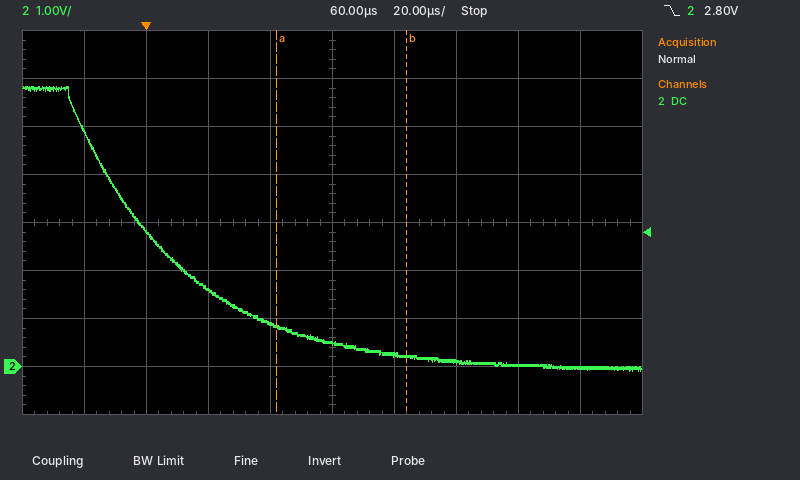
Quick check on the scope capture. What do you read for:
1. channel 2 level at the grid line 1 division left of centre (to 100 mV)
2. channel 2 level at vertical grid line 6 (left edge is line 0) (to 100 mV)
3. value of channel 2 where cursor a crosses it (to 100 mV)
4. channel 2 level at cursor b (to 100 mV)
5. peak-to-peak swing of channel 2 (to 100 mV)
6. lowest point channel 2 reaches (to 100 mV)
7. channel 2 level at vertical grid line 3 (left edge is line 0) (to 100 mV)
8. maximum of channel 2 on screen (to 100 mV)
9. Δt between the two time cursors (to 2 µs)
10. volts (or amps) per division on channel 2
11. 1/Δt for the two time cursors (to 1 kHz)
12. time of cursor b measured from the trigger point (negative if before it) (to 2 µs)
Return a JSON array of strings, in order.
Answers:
["900 mV", "200 mV", "800 mV", "200 mV", "5.9 V", "-100 mV", "1.6 V", "5.8 V", "42 µs", "1 V", "24 kHz", "+84 µs"]
